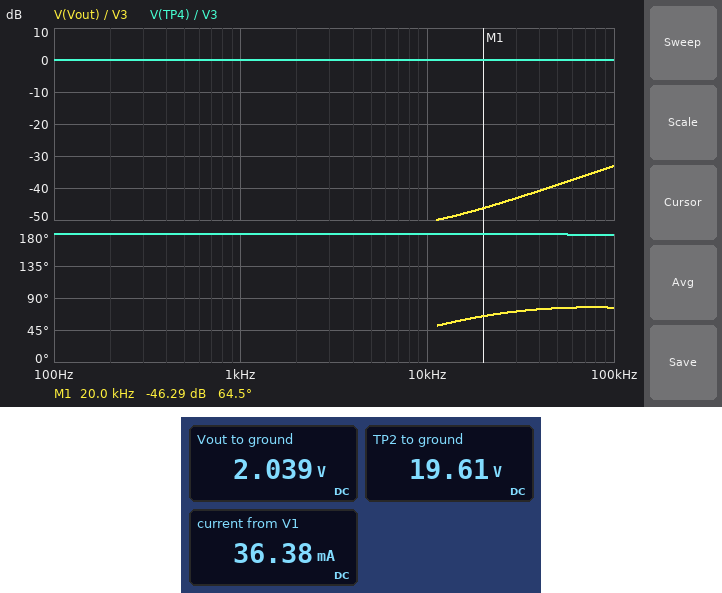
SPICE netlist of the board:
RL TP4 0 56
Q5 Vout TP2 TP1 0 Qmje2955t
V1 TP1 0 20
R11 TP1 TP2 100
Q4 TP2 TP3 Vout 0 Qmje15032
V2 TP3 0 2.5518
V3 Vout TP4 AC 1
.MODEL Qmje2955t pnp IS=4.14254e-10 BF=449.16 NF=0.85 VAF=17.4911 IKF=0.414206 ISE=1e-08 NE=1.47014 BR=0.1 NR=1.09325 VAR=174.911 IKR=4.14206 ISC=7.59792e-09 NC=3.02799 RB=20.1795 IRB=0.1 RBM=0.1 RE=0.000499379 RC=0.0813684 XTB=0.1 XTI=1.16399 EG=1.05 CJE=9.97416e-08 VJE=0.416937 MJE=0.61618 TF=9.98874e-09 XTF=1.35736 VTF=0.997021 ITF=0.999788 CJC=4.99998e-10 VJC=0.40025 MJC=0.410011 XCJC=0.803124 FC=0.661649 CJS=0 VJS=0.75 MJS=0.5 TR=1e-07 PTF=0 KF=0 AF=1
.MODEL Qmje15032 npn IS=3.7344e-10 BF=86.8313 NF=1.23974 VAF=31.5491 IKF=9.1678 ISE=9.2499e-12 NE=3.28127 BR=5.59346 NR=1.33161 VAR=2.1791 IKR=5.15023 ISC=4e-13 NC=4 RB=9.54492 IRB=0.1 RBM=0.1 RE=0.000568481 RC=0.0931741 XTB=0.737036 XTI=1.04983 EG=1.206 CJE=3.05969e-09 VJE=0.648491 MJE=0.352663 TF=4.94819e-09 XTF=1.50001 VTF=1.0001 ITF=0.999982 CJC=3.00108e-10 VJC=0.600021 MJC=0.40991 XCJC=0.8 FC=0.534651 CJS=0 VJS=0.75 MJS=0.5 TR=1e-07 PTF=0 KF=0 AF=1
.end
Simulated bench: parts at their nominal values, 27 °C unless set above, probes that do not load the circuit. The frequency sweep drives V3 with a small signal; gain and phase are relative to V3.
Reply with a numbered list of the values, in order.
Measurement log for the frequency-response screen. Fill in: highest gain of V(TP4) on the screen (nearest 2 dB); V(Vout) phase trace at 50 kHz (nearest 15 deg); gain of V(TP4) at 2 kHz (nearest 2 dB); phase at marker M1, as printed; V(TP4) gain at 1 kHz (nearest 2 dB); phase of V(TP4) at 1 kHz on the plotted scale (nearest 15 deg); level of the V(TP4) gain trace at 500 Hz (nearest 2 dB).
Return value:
1. 0 dB
2. 75 deg
3. 0 dB
4. 64.5 deg
5. 0 dB
6. 180 deg
7. 0 dB
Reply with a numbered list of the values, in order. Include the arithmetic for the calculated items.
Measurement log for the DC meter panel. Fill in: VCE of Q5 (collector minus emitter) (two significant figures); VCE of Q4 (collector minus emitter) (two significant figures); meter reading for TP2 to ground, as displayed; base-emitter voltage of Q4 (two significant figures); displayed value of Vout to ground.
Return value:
1. 2.039 V - 20 V = -18 V
2. 19.61 V - 2.039 V = 18 V
3. 19.61 V
4. 2.552 V - 2.039 V = 510 mV
5. 2.039 V
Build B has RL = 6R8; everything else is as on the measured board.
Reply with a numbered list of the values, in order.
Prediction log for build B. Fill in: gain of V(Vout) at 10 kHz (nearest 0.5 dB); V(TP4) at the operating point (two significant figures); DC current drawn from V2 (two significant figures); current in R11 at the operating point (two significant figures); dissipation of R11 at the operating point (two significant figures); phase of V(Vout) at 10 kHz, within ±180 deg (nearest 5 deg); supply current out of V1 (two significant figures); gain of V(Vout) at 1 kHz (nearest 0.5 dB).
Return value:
1. -45.0 dB
2. 2.0 V
3. 55 µA
4. 4.7 mA
5. 2.2 mW
6. 25 deg
7. 300 mA
8. -46.0 dB
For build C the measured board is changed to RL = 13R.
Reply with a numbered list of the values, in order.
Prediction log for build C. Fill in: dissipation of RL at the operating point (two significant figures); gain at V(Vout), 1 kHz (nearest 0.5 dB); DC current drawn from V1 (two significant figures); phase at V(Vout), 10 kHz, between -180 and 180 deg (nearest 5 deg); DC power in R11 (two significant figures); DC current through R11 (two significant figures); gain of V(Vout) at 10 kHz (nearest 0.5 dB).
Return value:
1. 320 mW
2. -49.5 dB
3. 160 mA
4. 35 deg
5. 1.9 mW
6. 4.4 mA
7. -48.0 dB
